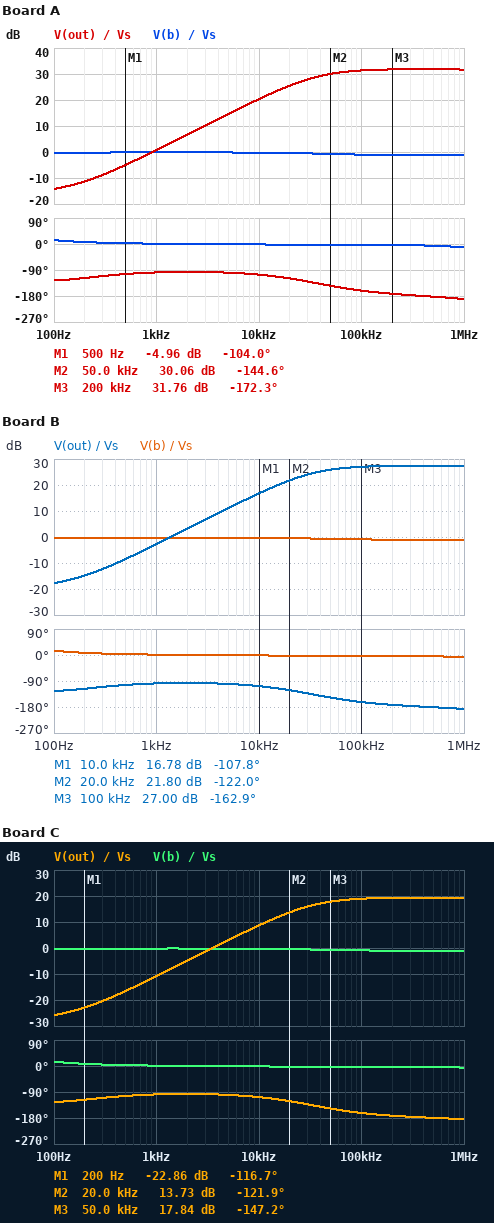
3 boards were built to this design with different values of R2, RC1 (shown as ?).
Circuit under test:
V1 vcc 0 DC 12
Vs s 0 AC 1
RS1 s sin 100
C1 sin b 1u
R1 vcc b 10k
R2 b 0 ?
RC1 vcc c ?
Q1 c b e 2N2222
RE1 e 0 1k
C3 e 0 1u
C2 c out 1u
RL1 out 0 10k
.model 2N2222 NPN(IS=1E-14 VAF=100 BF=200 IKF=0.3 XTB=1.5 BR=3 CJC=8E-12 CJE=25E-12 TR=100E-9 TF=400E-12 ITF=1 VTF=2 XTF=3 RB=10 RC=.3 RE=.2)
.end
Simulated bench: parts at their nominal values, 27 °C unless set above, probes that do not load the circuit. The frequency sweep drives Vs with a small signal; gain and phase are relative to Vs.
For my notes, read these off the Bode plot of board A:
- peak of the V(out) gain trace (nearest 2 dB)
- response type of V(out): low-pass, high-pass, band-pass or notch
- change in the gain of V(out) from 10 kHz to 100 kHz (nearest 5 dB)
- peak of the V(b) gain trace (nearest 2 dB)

32 dB
high-pass
10 dB
0 dB
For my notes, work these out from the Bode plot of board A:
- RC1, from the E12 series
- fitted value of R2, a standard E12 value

180 Ω
22 kΩ
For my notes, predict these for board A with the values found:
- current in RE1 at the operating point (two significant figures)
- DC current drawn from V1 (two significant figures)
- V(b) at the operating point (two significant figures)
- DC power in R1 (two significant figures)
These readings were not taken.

7.3 mA
7.7 mA
8.0 V
1.6 mW
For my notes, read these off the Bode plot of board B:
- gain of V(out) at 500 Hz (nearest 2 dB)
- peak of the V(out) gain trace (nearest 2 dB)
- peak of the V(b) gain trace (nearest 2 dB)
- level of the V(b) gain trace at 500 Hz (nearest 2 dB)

-8 dB
28 dB
0 dB
0 dB
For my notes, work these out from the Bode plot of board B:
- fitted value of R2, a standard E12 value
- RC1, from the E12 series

15 kΩ
120 Ω
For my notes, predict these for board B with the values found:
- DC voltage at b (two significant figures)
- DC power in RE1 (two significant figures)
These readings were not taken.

7.0 V
40 mW
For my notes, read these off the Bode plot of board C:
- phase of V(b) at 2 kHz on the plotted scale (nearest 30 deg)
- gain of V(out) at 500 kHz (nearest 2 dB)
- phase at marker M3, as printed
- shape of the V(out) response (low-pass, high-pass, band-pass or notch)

0 deg
20 dB
-147.2 deg
high-pass
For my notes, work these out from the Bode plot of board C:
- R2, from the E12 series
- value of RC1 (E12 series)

15 kΩ
47 Ω
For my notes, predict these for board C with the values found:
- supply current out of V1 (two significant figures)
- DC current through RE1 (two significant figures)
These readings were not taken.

6.8 mA
6.3 mA
